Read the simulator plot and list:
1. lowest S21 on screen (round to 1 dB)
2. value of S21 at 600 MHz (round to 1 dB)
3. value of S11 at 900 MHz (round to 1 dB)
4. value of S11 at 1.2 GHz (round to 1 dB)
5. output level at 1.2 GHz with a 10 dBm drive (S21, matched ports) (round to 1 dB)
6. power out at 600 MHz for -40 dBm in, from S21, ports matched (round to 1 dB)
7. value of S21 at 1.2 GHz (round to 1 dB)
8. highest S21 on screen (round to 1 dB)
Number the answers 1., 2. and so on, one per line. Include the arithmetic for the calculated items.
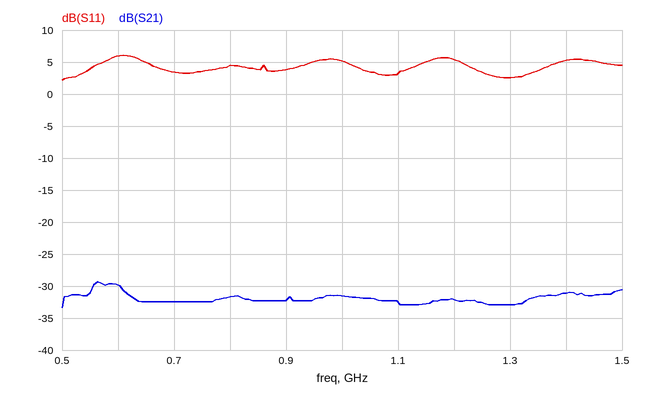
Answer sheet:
1. -33 dB
2. -30 dB
3. 4 dB
4. 5 dB
5. 10 dBm + (-32 dB) = -22 dBm
6. -40 dBm + (-30 dB) = -70 dBm
7. -32 dB
8. -29 dB
